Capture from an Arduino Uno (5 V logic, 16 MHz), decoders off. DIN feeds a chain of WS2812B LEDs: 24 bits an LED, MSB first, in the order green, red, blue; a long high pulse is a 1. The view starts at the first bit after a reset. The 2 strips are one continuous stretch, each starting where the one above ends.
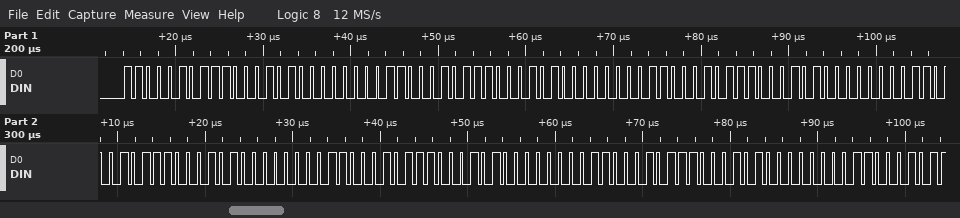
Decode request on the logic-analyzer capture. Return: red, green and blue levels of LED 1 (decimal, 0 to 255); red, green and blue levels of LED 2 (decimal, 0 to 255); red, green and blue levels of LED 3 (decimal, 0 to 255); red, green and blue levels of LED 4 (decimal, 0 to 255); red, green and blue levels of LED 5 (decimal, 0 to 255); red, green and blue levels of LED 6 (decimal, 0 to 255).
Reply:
197, 197, 0
197, 197, 0
197, 197, 0
197, 197, 0
197, 197, 0
197, 197, 0
